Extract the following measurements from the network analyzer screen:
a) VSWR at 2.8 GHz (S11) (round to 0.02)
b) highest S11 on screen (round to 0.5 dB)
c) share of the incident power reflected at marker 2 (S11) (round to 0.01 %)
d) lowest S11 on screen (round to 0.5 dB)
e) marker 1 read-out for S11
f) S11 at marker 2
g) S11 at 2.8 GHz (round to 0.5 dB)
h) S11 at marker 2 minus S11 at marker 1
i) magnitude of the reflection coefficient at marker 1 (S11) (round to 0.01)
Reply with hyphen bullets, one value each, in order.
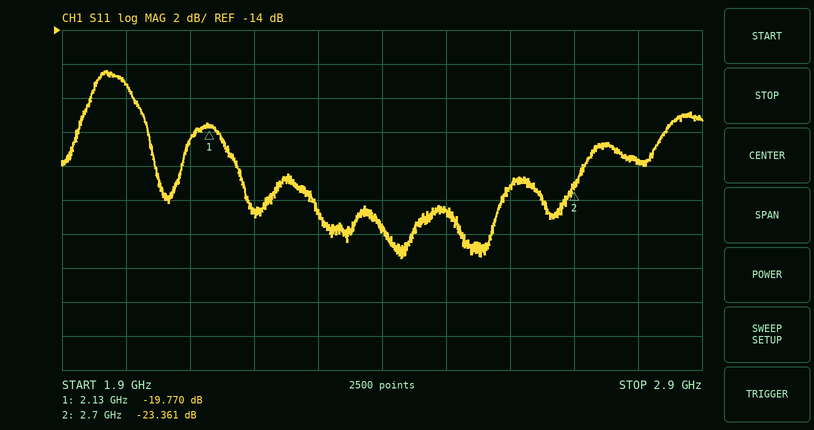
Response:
- 1.18
- -16.5 dB
- 0.46 %
- -27.5 dB
- -19.770 dB
- -23.361 dB
- -21.5 dB
- -3.591 dB
- 0.10
